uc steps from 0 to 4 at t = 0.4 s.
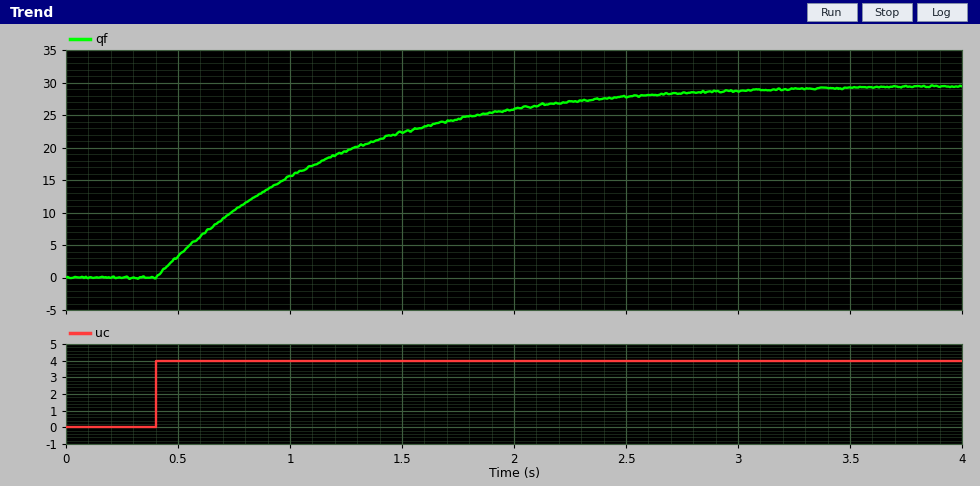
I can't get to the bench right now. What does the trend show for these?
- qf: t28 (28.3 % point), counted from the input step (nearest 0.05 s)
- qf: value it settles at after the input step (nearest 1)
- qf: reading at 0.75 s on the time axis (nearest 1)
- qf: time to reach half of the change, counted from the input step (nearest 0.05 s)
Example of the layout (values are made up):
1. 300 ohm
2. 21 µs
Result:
1. 0.25 s
2. 29
3. 10
4. 0.55 s
